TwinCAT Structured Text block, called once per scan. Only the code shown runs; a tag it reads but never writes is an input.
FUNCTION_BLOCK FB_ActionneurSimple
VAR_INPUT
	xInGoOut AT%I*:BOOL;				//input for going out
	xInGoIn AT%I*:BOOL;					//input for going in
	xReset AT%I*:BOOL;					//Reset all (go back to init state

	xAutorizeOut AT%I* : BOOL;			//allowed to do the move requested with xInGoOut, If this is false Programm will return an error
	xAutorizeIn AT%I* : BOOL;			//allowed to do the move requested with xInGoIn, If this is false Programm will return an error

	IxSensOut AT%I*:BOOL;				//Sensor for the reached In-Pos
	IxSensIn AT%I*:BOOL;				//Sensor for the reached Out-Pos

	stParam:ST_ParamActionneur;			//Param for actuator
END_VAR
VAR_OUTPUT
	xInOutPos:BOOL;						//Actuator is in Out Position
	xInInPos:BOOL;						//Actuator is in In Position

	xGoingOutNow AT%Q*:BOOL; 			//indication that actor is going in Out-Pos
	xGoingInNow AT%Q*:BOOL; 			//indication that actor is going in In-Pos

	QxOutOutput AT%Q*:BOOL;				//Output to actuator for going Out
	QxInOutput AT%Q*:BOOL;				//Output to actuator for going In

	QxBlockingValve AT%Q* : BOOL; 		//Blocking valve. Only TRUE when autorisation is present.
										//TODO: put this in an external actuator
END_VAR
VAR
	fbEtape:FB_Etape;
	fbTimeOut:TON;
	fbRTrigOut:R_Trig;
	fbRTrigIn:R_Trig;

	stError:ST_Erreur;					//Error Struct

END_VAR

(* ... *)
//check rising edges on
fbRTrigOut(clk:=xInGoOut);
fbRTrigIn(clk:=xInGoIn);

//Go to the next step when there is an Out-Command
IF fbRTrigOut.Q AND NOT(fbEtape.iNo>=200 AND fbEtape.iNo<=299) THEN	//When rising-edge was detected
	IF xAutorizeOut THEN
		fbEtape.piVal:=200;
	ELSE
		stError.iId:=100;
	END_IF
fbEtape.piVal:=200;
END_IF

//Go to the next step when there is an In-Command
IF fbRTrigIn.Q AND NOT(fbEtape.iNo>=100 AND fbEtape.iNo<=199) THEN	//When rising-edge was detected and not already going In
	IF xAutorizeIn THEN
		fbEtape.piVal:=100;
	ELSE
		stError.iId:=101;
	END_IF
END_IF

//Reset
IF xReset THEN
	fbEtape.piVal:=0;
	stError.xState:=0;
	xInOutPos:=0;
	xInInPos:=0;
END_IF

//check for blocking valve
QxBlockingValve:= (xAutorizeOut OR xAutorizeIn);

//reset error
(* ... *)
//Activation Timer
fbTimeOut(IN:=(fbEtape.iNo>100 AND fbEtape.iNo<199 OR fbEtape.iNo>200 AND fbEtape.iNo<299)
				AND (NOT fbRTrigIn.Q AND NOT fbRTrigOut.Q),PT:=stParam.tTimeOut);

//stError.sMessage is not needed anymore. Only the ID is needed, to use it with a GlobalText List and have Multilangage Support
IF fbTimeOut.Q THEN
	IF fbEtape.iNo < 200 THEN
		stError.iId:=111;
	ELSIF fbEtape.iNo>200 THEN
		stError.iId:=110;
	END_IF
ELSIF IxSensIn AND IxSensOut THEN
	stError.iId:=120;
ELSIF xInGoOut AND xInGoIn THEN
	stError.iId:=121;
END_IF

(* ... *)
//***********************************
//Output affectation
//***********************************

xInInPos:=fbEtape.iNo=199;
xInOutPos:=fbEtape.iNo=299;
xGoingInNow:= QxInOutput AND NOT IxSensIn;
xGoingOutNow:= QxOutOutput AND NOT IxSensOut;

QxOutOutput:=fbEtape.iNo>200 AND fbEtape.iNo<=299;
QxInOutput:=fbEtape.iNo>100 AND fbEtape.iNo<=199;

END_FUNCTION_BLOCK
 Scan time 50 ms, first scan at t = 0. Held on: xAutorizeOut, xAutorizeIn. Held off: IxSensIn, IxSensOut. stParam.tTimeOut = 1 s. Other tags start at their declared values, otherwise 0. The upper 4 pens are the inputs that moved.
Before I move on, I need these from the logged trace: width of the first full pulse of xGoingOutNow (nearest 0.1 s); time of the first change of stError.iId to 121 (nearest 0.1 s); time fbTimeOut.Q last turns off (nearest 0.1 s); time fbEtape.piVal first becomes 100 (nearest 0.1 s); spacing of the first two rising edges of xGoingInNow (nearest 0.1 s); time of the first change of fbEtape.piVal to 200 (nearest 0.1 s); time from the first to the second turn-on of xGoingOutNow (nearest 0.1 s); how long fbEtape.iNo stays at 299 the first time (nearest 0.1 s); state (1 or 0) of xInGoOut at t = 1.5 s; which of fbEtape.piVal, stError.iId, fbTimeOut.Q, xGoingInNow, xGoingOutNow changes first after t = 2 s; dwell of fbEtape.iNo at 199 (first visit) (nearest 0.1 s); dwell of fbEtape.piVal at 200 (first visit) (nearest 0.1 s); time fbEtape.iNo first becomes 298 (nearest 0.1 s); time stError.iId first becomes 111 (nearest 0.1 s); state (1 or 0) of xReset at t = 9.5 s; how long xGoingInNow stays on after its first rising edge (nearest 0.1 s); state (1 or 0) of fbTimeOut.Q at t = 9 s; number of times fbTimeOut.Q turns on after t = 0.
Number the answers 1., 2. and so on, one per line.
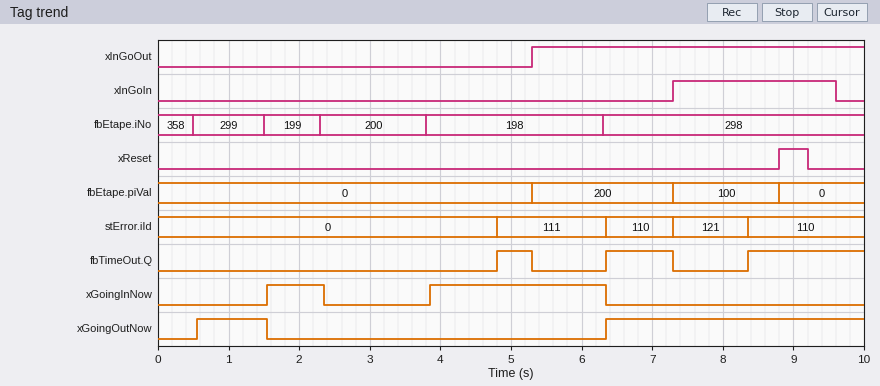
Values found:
1. 1.0 s
2. 7.3 s
3. 7.3 s
4. 7.3 s
5. 2.3 s
6. 5.3 s
7. 5.8 s
8. 1.0 s
9. 0
10. xGoingInNow
11. 0.8 s
12. 2.0 s
13. 6.3 s
14. 4.8 s
15. 0
16. 0.8 s
17. 1
18. 3
